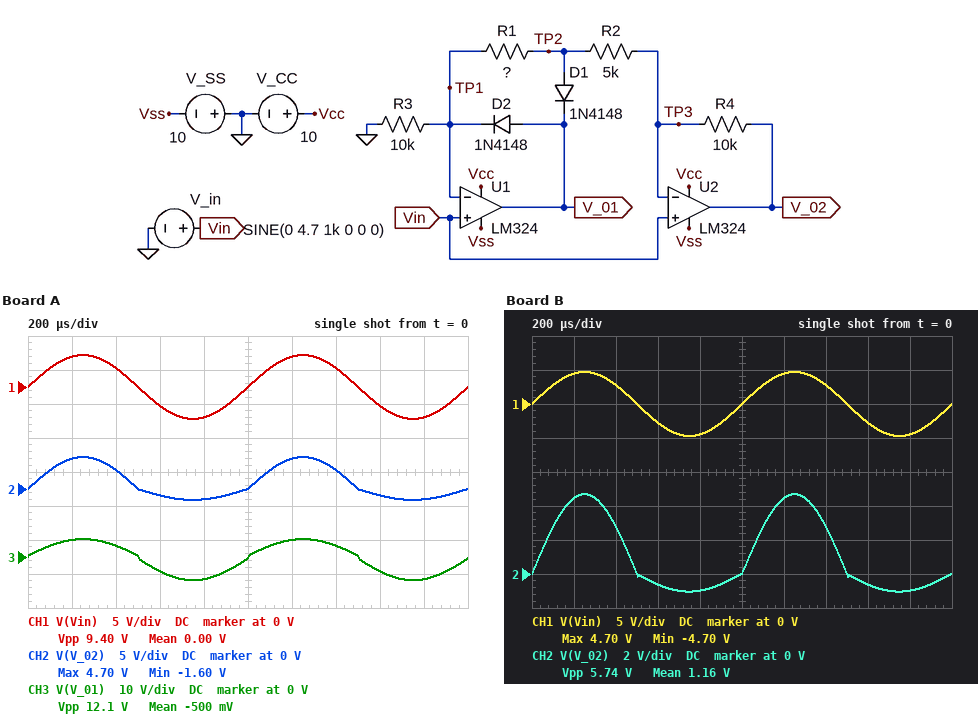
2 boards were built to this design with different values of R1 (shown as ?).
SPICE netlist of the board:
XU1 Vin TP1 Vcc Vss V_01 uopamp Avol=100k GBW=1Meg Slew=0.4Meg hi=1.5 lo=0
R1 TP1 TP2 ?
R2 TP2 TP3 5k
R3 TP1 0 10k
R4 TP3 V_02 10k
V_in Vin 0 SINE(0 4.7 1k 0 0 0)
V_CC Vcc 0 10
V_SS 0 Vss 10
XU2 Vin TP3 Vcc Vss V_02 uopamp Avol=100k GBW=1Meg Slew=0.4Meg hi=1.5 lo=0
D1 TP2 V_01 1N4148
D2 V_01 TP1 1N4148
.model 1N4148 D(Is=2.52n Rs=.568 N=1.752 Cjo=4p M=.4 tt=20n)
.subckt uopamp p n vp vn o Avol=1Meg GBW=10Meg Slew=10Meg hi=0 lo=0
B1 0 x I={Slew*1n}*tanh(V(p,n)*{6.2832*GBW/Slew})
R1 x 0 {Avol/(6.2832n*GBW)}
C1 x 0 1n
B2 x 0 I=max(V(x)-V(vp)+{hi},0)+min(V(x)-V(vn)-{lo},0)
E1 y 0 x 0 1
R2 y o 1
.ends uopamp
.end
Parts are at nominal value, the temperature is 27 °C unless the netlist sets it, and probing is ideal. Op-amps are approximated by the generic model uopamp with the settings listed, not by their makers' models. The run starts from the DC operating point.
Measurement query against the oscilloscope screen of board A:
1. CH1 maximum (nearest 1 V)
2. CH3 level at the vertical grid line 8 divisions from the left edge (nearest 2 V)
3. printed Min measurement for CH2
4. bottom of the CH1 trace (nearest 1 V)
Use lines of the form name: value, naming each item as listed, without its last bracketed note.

CH1 maximum: 5 V
CH3 level at the vertical grid line 8 divisions from the left edge: -4 V
printed Min measurement for CH2: -1.60 V
bottom of the CH1 trace: -5 V
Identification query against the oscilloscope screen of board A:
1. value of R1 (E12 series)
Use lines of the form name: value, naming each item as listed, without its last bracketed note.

value of R1: 3.3 kΩ
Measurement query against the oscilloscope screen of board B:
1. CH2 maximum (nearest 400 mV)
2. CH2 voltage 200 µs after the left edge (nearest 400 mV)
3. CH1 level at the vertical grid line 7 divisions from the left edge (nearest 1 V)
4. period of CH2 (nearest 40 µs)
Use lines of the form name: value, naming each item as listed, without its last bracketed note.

CH2 maximum: 4.8 V
CH2 voltage 200 µs after the left edge: 4.4 V
CH1 level at the vertical grid line 7 divisions from the left edge: 3 V
period of CH2: 1.00 ms
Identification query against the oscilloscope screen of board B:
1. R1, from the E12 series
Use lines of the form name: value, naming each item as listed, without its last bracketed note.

R1, from the E12 series: 3.9 kΩ
